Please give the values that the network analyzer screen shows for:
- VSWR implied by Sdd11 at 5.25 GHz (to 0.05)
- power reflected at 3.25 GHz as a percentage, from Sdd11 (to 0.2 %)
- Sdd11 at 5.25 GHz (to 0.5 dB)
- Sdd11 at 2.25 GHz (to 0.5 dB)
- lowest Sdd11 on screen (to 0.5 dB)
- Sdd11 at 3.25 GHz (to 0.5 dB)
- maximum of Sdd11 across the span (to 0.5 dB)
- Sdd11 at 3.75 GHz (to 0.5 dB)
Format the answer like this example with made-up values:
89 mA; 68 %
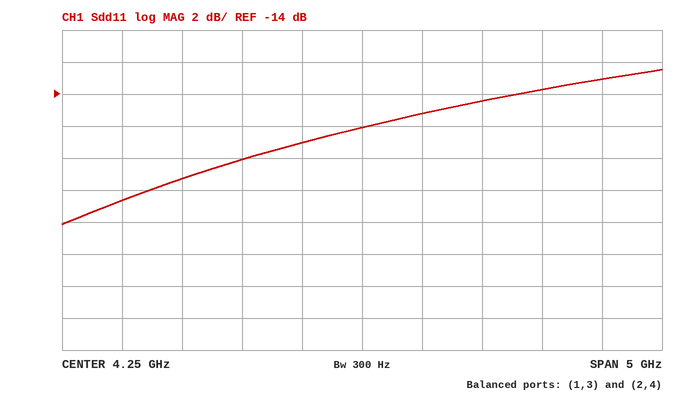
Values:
1.45; 1.6 %; -14.5 dB; -20.5 dB; -22.0 dB; -18.0 dB; -12.5 dB; -17.0 dB
